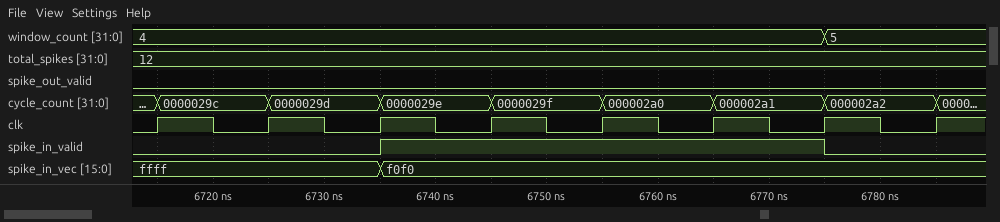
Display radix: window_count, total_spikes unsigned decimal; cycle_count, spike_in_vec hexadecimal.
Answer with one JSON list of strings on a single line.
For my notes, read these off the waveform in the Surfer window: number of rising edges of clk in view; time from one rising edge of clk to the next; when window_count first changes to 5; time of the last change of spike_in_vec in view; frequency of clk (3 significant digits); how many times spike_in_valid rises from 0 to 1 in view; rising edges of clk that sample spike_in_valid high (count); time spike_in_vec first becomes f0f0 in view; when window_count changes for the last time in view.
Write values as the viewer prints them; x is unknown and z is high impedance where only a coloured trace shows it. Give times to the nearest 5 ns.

["8", "10 ns", "6775 ns", "6735 ns", "100 MHz", "1", "4", "6735 ns", "6775 ns"]
